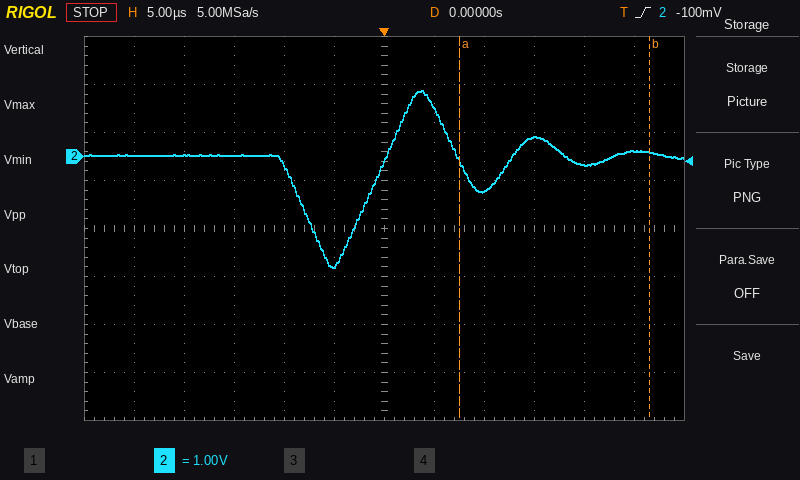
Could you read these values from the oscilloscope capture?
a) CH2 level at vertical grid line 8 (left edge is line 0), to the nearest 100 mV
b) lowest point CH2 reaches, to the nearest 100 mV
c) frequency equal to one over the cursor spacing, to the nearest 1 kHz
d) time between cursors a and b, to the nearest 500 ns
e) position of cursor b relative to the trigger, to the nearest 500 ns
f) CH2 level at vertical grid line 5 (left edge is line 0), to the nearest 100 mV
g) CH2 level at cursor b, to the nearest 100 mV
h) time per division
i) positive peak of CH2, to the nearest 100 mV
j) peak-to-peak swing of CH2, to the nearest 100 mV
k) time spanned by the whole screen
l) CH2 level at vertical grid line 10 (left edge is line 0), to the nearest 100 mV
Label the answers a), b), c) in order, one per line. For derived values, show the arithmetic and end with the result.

a) -700 mV
b) -2.3 V
c) 1 / 19.0 µs ≈ 53 kHz
d) 19.0 µs
e) +26.5 µs
f) -2.3 V
g) 100 mV
h) 5 µs
i) 1.4 V
j) 1.4 V − (-2.3 V) = 3.7 V
k) 60 µs
l) -200 mV
